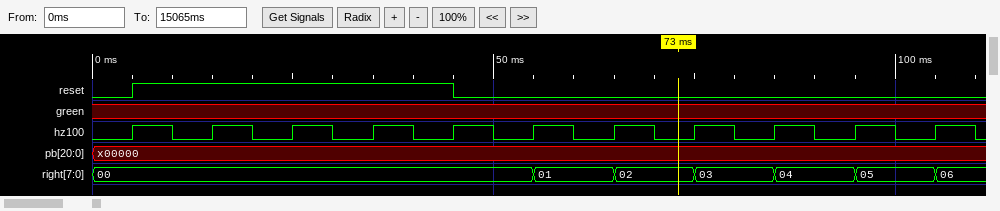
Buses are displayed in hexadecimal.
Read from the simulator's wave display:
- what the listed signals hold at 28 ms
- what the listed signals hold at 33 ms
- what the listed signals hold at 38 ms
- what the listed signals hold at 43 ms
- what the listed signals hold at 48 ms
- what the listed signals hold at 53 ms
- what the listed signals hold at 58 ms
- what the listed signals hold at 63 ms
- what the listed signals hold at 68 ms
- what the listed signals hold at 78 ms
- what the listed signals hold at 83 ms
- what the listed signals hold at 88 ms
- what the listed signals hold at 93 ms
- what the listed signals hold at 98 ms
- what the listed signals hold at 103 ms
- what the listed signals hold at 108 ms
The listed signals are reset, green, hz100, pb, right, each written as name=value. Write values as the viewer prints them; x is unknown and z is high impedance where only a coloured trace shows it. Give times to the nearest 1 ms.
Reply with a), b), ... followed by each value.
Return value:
a) reset=1, green=x, hz100=1, pb=x00000, right=00
b) reset=1, green=x, hz100=0, pb=x00000, right=00
c) reset=1, green=x, hz100=1, pb=x00000, right=00
d) reset=1, green=x, hz100=0, pb=x00000, right=00
e) reset=0, green=x, hz100=1, pb=x00000, right=00
f) reset=0, green=x, hz100=0, pb=x00000, right=00
g) reset=0, green=x, hz100=1, pb=x00000, right=01
h) reset=0, green=x, hz100=0, pb=x00000, right=01
i) reset=0, green=x, hz100=1, pb=x00000, right=02
j) reset=0, green=x, hz100=1, pb=x00000, right=03
k) reset=0, green=x, hz100=0, pb=x00000, right=03
l) reset=0, green=x, hz100=1, pb=x00000, right=04
m) reset=0, green=x, hz100=0, pb=x00000, right=04
n) reset=0, green=x, hz100=1, pb=x00000, right=05
o) reset=0, green=x, hz100=0, pb=x00000, right=05
p) reset=0, green=x, hz100=1, pb=x00000, right=06
